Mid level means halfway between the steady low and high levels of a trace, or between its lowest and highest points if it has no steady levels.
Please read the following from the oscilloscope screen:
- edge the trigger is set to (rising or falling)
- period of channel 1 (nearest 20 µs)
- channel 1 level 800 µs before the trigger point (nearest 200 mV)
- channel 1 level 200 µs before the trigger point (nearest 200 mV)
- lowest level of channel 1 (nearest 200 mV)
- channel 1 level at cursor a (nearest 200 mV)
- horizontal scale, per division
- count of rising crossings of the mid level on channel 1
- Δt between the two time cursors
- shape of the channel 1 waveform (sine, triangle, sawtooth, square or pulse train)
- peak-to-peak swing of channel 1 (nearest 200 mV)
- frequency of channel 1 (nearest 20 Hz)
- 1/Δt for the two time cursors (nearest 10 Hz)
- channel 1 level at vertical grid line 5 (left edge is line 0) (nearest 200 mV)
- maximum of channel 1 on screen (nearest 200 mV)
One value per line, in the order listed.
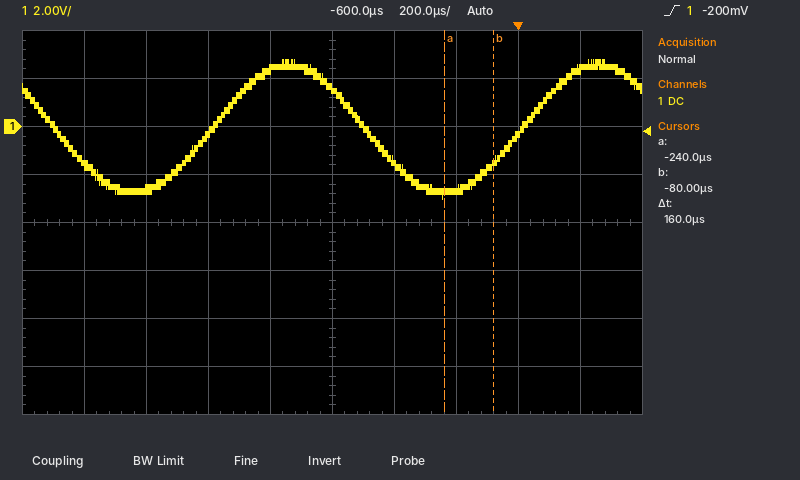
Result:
rising
1.00 ms
2.4 V
-2.6 V
-3.0 V
-2.8 V
200 µs
2
160 µs
sine
5.8 V
1.00 kHz
6.25 kHz
1.6 V
2.8 V
